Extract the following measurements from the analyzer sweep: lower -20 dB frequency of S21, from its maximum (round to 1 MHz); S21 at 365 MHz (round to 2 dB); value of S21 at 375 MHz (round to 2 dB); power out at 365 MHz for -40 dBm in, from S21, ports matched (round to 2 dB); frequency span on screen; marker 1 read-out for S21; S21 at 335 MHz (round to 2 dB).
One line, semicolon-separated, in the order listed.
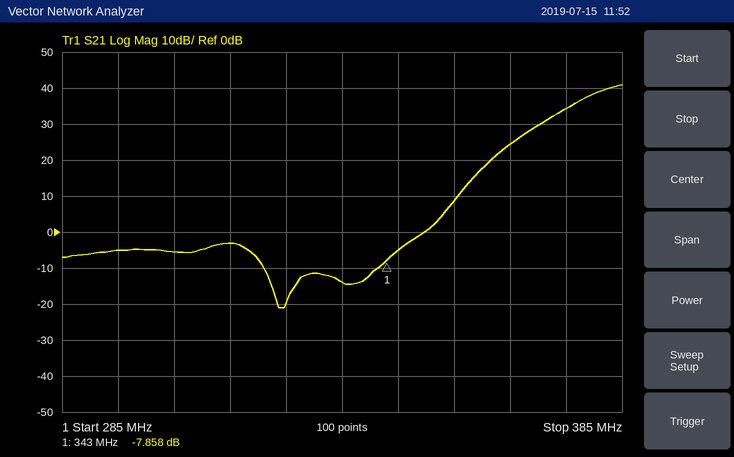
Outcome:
362 MHz; 24 dB; 34 dB; -16 dBm; 100 MHz; -7.858 dB; -14 dB
